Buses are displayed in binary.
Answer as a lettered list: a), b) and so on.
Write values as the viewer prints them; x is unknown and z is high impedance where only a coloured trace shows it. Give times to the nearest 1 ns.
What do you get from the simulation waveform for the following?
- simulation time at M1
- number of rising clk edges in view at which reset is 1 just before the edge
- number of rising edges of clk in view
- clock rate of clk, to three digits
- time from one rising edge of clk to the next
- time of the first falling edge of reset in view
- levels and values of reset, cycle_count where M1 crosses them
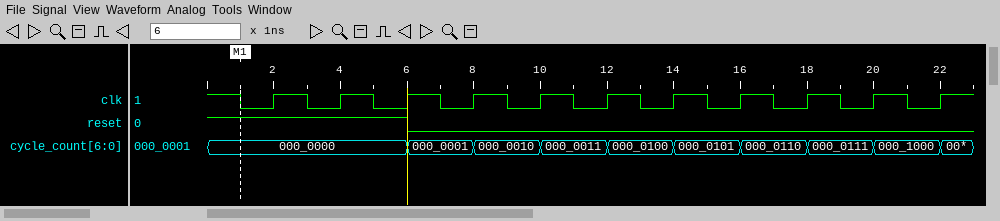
a) 1 ns
b) 3
c) 11
d) 500 MHz
e) 2 ns
f) 6 ns
g) reset=1, cycle_count=000_0000
